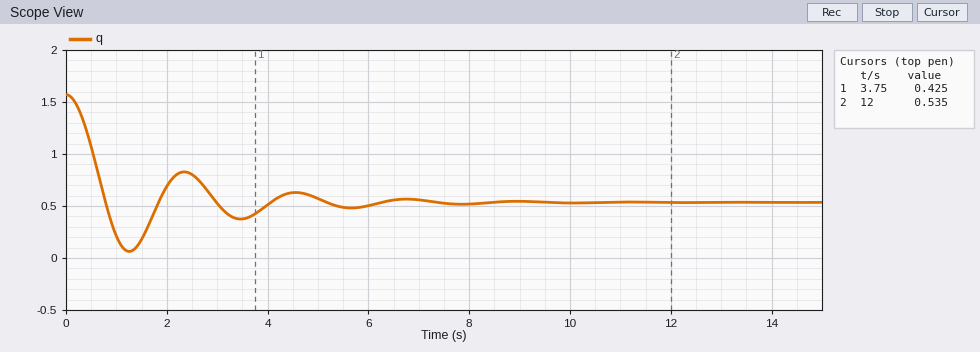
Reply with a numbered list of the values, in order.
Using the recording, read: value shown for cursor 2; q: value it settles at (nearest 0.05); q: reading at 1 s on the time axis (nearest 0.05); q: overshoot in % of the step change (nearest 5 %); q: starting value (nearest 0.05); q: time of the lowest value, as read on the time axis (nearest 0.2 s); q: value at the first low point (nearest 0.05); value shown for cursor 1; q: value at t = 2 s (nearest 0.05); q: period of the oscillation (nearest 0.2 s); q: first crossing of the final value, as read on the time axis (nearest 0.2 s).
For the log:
1. 0.535
2. 0.55
3. 0.20
4. 45 %
5. 1.55
6. 1.2 s
7. 0.05
8. 0.425
9. 0.70
10. 2.2 s
11. 0.8 s
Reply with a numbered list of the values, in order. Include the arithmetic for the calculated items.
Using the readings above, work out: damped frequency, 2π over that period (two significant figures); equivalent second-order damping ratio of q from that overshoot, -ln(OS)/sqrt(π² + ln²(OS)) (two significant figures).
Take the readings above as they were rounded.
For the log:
1. 2π / 2.2 = 2.9 rad/s
2. ln(0.45) = -0.799; 0.799 / sqrt(9.870 + 0.638) = 0.25
